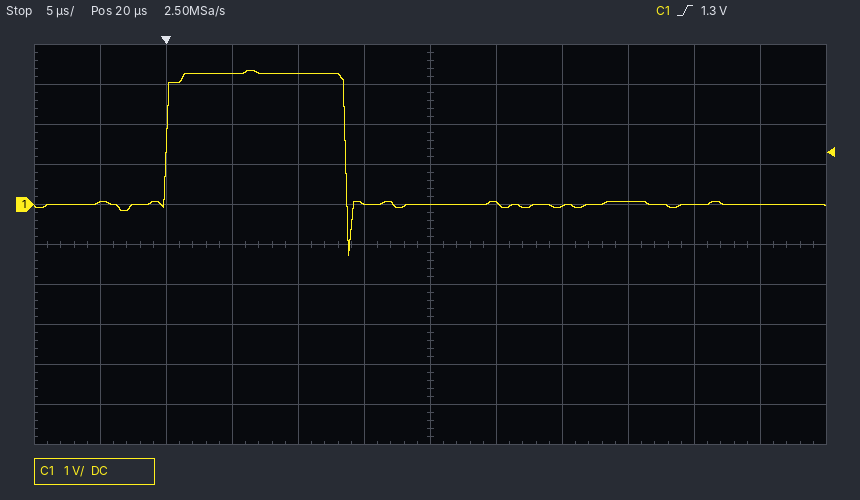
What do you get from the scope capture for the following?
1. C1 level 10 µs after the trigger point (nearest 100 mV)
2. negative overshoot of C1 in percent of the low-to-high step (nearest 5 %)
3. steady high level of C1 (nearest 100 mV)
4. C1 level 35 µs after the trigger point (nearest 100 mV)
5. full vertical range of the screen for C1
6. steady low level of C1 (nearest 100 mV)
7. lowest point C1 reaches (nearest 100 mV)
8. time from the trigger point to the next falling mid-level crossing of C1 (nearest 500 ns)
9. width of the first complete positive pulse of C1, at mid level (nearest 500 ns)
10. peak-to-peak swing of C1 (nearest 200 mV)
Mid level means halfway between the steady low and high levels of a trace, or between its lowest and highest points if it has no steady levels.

3.3 V
40 %
3.3 V
100 mV
10 V
0.0 V
-1.3 V
13.5 µs
13.5 µs
4.6 V
